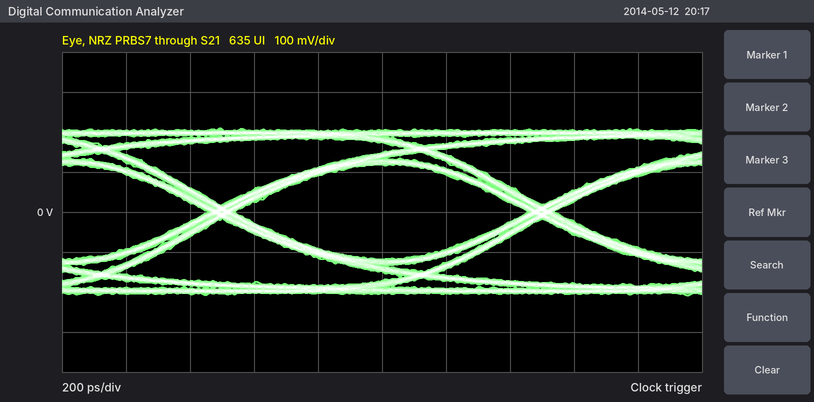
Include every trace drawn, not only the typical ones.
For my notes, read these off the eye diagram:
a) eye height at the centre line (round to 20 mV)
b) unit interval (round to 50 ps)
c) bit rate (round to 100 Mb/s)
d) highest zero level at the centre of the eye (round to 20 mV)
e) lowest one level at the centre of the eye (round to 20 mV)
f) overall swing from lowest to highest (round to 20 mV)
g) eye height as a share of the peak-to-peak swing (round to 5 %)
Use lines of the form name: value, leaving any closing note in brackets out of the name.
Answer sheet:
eye height at the centre line: 240 mV
unit interval: 1.00 ns
bit rate: 1.0 Gb/s
highest zero level at the centre of the eye: -120 mV
lowest one level at the centre of the eye: 120 mV
overall swing from lowest to highest: 420 mV
eye height as a share of the peak-to-peak swing: 55 %
